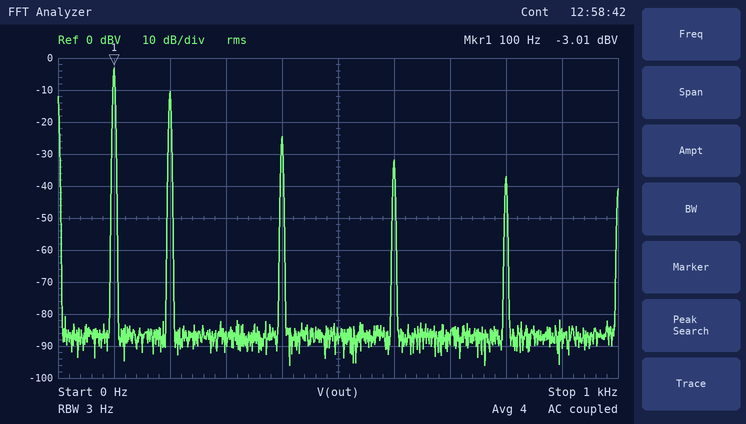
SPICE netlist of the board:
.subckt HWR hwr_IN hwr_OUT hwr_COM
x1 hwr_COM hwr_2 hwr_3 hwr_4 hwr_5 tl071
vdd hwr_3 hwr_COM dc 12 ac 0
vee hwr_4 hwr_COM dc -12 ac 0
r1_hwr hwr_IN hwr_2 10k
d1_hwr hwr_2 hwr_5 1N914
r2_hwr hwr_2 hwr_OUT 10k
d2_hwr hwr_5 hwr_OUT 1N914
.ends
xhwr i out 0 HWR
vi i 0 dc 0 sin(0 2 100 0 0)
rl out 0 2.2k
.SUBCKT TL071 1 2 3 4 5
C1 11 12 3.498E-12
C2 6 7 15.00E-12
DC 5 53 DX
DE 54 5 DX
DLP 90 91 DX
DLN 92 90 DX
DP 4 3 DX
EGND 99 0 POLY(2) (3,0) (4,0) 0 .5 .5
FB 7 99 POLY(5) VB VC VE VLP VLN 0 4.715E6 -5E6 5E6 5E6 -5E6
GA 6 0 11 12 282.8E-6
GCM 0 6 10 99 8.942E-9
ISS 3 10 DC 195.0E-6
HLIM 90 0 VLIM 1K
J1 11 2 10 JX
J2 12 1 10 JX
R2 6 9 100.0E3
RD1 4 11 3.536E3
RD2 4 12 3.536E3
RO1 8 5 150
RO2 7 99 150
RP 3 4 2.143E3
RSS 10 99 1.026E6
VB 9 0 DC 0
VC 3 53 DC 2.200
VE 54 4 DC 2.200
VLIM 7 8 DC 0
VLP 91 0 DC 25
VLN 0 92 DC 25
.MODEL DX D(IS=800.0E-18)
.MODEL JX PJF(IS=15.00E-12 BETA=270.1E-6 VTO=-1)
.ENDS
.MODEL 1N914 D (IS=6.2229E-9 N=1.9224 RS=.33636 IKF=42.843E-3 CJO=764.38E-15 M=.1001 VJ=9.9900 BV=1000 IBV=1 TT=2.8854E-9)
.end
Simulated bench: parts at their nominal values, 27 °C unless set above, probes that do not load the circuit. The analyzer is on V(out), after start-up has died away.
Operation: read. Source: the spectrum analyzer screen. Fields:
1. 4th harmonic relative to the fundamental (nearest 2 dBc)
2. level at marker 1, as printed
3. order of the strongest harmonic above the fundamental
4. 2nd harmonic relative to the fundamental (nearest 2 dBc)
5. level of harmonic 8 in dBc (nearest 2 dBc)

-22 dBc
-3.01 dBV
2
-8 dBc
-34 dBc
